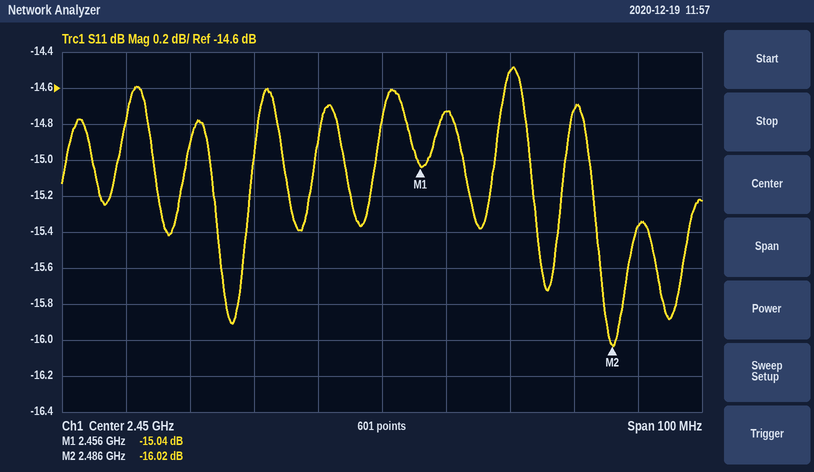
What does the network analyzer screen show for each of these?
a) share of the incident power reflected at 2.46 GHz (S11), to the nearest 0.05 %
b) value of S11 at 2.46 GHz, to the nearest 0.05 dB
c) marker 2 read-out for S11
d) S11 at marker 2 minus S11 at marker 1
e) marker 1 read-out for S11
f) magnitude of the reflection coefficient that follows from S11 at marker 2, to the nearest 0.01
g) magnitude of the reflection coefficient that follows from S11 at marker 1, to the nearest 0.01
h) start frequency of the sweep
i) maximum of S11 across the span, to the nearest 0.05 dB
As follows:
3.35 %
-14.75 dB
-16.02 dB
-0.98 dB
-15.04 dB
0.16
0.18
2.4 GHz
-14.50 dB
